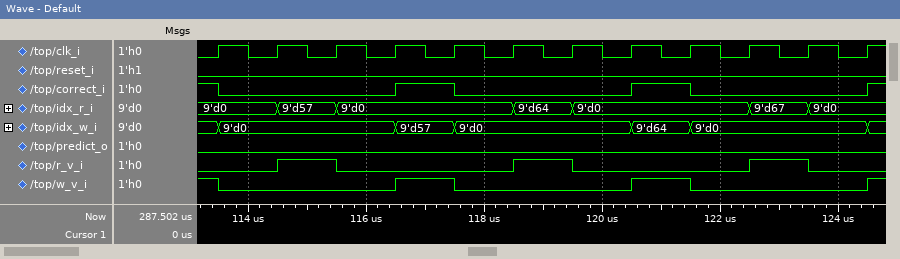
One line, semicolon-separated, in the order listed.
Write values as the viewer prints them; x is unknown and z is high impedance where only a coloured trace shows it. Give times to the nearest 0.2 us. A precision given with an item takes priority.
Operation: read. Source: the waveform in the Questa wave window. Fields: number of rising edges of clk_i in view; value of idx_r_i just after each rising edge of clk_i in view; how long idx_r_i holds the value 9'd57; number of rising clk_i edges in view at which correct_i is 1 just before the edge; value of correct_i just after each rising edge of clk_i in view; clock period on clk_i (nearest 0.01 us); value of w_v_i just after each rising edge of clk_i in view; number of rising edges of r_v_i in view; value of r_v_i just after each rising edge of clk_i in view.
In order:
12; 9'd0, 9'd57, 9'd0, 9'd0, 9'd0, 9'd64, 9'd0, 9'd0, 9'd0, 9'd67, 9'd0, 9'd0; 1 us; 3; 0 0 0 1 0 0 0 1 0 0 0 1; 1 us; 0 0 0 1 0 0 0 1 0 0 0 1; 3; 0 1 0 0 0 1 0 0 0 1 0 0
